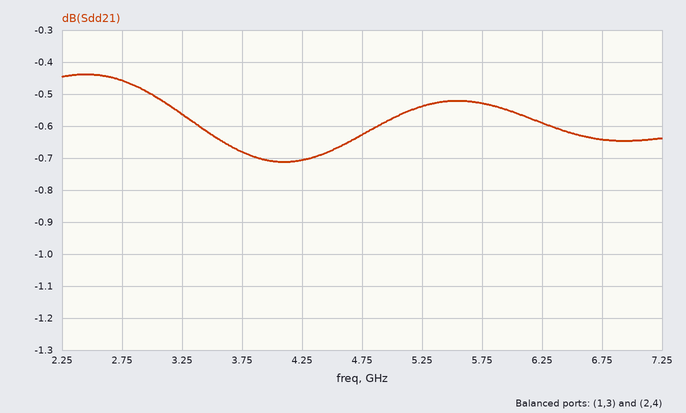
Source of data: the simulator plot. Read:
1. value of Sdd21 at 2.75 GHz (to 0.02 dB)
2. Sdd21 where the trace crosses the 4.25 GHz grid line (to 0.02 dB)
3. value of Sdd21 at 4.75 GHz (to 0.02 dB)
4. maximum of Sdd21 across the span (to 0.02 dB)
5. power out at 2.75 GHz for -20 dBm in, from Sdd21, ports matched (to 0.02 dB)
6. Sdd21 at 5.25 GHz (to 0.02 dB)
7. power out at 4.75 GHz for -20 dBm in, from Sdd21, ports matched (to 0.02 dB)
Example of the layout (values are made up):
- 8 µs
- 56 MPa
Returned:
- -0.46 dB
- -0.70 dB
- -0.62 dB
- -0.44 dB
- -20.46 dBm
- -0.54 dB
- -20.62 dBm
